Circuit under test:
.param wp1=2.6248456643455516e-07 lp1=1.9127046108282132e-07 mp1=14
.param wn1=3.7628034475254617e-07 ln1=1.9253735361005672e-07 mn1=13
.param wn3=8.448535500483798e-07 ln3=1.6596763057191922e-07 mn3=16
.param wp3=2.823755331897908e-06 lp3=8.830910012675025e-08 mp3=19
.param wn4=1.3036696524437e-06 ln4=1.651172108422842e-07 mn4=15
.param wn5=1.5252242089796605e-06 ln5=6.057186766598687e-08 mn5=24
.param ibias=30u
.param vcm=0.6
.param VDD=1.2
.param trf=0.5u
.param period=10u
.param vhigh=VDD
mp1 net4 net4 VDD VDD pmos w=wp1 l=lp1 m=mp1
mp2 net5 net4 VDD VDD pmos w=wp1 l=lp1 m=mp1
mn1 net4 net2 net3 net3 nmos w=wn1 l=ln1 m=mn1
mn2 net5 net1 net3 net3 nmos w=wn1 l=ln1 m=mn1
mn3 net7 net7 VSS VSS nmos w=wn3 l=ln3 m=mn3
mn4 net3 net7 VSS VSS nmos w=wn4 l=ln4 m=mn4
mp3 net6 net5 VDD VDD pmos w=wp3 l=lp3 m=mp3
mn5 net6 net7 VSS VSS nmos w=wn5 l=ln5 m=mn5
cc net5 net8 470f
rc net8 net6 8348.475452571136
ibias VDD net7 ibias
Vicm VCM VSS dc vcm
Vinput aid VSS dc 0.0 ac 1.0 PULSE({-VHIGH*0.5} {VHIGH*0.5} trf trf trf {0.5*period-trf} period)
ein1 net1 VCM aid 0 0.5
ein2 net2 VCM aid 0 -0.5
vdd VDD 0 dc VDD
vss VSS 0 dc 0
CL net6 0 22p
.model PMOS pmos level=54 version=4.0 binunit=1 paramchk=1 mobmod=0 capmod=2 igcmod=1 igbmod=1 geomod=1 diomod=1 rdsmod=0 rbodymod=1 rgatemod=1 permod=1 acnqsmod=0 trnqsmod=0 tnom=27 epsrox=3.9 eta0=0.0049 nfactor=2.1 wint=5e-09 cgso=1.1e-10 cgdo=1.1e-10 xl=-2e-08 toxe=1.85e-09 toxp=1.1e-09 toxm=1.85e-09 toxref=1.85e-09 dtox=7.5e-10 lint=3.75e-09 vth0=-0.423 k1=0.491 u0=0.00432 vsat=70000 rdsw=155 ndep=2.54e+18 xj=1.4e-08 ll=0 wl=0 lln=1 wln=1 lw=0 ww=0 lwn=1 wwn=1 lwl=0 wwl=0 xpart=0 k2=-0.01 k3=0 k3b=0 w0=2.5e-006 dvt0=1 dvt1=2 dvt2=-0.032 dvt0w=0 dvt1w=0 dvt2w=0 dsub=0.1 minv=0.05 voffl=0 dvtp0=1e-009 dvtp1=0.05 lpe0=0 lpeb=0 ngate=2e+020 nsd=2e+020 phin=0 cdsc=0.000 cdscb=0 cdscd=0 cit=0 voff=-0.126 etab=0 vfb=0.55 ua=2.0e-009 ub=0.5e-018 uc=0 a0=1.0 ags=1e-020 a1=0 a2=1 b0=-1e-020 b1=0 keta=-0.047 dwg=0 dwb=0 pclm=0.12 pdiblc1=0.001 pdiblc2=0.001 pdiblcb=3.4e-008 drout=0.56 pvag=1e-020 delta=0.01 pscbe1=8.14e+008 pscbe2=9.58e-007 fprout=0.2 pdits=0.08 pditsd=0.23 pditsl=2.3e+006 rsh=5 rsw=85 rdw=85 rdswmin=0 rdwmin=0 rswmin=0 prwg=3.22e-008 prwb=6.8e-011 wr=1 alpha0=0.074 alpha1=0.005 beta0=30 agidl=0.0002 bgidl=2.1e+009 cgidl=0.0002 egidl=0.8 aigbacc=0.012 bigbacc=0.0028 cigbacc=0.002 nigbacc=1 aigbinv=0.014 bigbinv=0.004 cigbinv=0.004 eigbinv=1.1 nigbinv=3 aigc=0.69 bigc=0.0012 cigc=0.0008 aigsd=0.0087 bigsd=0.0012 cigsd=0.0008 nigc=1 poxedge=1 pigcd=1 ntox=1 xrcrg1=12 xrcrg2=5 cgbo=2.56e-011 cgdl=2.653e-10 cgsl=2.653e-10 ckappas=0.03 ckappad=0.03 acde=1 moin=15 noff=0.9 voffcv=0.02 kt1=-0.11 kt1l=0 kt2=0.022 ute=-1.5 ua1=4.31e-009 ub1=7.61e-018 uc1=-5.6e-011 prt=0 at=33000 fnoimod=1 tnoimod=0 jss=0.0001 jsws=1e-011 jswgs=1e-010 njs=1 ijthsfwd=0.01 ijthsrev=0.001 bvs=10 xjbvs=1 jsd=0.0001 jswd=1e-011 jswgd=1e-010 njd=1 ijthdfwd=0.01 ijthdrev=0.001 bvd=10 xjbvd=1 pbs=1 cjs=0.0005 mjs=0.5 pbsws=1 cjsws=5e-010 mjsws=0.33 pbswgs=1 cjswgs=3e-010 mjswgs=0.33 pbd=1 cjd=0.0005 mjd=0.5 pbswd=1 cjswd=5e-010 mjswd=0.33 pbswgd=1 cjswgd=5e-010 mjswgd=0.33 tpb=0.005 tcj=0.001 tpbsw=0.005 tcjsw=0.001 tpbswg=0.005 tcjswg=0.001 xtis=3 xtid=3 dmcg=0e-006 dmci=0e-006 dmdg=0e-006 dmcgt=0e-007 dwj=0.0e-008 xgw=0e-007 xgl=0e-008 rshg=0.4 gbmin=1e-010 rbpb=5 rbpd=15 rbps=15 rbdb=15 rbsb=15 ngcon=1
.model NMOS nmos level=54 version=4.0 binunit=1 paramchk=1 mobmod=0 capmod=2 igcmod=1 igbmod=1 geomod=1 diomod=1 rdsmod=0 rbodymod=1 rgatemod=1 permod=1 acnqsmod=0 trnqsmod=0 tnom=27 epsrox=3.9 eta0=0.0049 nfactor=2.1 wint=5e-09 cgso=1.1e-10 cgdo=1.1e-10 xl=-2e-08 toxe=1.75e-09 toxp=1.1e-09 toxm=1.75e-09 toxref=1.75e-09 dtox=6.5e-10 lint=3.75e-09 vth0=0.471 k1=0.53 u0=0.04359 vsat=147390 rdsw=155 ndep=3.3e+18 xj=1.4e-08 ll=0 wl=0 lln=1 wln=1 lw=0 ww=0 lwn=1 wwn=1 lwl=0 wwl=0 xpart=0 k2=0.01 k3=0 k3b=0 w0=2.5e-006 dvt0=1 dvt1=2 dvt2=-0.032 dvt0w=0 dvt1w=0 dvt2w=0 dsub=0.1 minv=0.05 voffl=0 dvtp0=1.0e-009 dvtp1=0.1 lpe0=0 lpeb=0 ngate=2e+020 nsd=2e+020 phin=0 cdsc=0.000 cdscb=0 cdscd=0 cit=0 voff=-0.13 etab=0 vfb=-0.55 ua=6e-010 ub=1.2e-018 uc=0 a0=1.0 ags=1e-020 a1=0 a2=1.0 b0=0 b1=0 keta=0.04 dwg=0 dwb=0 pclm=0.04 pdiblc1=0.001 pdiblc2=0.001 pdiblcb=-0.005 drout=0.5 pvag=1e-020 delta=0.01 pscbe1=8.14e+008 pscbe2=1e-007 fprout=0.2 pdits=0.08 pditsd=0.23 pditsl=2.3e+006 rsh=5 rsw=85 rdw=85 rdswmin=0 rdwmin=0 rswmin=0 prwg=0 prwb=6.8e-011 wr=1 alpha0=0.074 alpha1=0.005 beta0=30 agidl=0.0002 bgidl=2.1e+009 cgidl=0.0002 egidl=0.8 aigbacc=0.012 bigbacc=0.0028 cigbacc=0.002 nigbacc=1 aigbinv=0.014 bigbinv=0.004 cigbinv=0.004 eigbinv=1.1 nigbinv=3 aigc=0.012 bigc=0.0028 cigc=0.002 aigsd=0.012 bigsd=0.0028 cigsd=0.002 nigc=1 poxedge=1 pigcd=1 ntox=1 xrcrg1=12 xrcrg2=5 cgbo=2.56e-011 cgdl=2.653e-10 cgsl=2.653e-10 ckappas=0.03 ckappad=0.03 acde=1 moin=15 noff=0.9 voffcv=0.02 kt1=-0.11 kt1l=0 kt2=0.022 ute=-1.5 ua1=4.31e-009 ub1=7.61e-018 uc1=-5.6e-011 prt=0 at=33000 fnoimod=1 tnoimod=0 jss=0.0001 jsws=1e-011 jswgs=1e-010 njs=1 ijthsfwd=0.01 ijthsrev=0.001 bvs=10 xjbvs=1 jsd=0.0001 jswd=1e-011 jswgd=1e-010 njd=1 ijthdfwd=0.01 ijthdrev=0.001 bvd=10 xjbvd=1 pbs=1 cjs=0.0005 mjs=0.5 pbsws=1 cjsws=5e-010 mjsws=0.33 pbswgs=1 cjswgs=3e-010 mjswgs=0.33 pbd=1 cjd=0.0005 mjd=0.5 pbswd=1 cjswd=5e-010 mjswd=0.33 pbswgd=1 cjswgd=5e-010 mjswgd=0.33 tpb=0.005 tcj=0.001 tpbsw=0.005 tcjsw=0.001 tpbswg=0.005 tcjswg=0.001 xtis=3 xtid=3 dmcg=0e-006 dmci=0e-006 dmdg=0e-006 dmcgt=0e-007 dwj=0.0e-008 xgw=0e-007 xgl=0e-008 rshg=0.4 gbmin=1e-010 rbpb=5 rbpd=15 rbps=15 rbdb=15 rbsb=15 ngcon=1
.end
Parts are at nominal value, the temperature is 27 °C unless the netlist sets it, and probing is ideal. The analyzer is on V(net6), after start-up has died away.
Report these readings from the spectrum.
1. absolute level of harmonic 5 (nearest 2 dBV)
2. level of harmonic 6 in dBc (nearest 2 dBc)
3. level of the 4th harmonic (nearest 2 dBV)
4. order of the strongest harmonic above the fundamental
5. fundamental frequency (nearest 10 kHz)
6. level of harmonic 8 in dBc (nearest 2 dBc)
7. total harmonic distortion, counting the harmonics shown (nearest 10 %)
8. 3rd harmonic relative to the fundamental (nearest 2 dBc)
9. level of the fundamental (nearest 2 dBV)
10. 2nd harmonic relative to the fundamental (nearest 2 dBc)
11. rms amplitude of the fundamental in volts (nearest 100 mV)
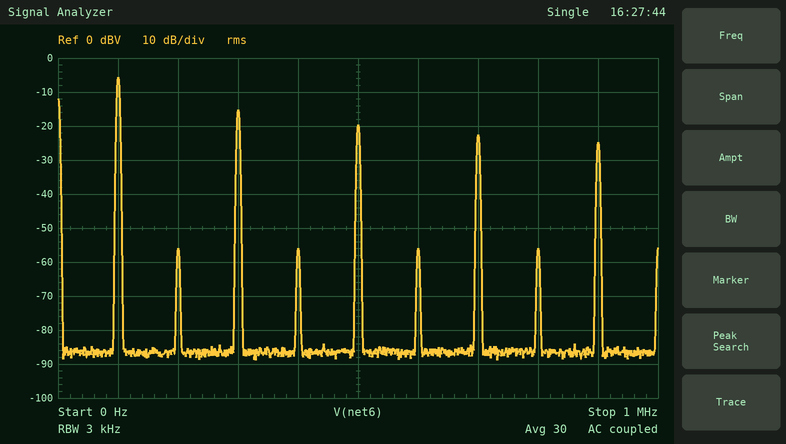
-20 dBV
-50 dBc
-56 dBV
3
100 kHz
-50 dBc
40 %
-10 dBc
-6 dBV
-50 dBc
500 mV
